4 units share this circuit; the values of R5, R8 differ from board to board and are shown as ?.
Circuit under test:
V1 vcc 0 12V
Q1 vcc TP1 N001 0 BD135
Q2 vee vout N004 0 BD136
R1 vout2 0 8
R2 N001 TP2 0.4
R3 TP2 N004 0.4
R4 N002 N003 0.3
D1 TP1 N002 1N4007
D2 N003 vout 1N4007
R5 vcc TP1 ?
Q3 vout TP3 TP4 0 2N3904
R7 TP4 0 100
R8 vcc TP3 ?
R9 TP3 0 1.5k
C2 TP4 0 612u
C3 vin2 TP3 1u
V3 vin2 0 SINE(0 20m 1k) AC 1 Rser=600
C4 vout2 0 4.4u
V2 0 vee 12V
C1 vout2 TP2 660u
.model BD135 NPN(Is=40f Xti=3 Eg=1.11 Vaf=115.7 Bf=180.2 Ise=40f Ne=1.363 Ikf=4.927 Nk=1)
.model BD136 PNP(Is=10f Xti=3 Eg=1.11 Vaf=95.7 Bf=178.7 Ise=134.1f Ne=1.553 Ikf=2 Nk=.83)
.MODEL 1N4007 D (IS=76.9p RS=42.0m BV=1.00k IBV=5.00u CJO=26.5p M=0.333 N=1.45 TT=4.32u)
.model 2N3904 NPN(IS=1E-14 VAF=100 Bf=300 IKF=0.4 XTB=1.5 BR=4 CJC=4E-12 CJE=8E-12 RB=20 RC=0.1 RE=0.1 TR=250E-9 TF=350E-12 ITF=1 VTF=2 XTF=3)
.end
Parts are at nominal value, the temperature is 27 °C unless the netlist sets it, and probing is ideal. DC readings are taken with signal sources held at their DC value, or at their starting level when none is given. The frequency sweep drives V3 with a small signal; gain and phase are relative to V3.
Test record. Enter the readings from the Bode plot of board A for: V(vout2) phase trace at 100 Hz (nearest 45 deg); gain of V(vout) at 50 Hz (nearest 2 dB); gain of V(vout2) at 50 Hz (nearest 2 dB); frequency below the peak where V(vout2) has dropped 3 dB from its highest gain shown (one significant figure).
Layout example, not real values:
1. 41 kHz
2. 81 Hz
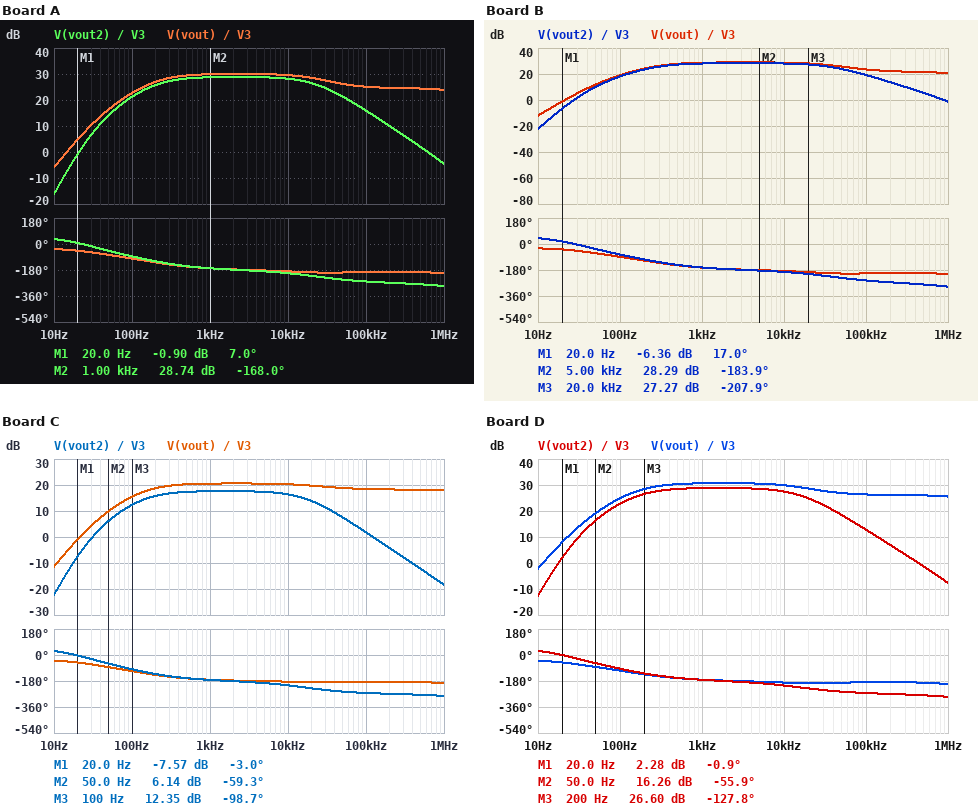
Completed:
1. -90 deg
2. 16 dB
3. 14 dB
4. 200 Hz
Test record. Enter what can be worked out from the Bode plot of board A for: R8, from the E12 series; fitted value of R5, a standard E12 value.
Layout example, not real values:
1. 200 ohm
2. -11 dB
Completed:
1. 6.8 kΩ
2. 180 Ω
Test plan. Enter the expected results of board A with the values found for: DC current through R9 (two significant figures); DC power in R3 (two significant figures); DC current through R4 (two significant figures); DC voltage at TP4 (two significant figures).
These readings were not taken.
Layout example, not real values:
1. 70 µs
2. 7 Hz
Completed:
1. 1.4 mA
2. 120 µW
3. 14 mA
4. 1.4 V
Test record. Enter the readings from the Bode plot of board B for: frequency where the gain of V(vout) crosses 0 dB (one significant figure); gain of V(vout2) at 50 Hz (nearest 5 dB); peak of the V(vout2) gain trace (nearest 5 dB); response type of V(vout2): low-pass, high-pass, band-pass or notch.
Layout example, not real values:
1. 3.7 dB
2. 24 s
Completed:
1. 20 Hz
2. 10 dB
3. 30 dB
4. band-pass
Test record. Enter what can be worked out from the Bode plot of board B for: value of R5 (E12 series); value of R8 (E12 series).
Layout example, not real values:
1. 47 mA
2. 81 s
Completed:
1. 120 Ω
2. 2.2 kΩ
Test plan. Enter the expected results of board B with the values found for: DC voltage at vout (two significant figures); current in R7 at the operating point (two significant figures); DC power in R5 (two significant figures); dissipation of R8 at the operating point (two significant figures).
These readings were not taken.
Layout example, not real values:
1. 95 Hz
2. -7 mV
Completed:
1. 5.7 V
2. 40 mA
3. 190 mW
4. 24 mW
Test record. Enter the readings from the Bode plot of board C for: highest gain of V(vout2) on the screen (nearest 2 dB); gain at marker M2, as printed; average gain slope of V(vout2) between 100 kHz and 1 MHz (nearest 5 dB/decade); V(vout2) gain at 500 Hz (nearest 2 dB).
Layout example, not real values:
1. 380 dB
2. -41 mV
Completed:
1. 18 dB
2. 6.14 dB
3. -20 dB/decade
4. 18 dB
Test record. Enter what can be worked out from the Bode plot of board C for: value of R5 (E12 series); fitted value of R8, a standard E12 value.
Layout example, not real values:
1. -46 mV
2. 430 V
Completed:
1. 82 Ω
2. 12 kΩ
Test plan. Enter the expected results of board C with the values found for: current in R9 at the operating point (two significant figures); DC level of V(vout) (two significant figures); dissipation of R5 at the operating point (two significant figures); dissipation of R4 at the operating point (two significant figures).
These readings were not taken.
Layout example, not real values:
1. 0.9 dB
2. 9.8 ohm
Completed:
1. 870 µA
2. 10 V
3. 3.0 mW
4. 11 µW
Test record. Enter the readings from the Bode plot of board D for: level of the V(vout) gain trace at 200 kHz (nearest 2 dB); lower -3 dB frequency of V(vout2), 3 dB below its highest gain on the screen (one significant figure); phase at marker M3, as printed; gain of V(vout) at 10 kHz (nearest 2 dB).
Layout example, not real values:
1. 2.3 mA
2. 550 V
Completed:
1. 26 dB
2. 200 Hz
3. -127.8 deg
4. 30 dB
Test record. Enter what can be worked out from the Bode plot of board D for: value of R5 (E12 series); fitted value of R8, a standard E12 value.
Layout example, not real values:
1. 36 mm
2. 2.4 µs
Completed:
1. 270 Ω
2. 10 kΩ
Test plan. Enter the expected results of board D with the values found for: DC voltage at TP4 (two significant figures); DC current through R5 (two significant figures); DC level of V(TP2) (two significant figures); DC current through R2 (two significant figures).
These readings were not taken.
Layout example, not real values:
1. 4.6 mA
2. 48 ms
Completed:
1. 820 mV
2. 8.2 mA
3. 9.1 V
4. 8.9 mA
